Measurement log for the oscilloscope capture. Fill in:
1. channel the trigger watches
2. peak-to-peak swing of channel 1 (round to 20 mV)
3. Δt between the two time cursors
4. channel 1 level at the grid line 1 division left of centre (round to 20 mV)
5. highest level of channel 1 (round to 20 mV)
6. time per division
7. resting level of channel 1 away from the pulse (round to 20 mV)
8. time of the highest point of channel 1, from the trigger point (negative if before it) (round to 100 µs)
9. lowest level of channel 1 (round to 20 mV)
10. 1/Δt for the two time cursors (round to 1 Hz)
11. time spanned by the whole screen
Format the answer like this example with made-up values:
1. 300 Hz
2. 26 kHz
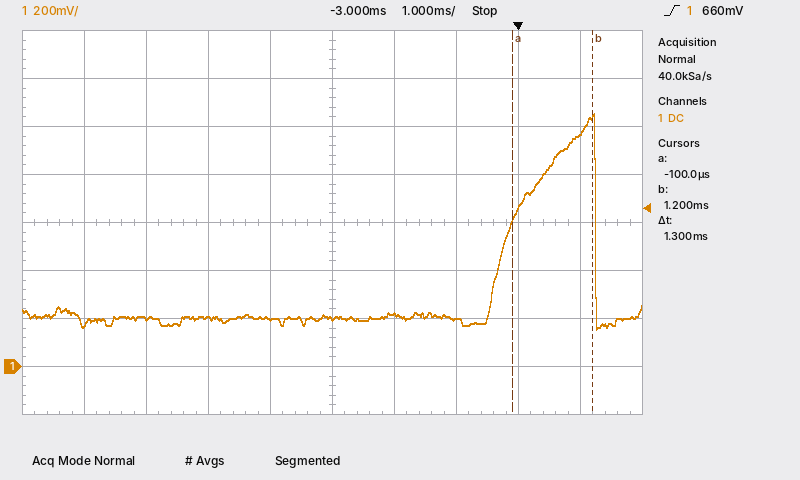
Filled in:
1. channel 1
2. 900 mV
3. 1.3 ms
4. 200 mV
5. 1.06 V
6. 1 ms
7. 200 mV
8. +1.2 ms
9. 160 mV
10. 769 Hz
11. 10 ms
